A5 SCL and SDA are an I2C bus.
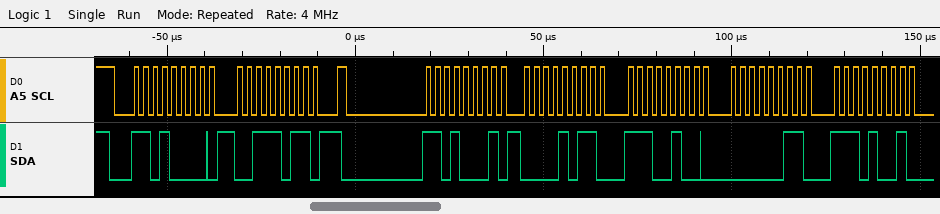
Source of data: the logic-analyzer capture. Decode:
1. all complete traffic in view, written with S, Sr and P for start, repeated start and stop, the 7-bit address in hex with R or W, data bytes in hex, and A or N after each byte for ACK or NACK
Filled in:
S 68W A 3B A Sr 68R A 0B A E4 A 03 A E9 A
